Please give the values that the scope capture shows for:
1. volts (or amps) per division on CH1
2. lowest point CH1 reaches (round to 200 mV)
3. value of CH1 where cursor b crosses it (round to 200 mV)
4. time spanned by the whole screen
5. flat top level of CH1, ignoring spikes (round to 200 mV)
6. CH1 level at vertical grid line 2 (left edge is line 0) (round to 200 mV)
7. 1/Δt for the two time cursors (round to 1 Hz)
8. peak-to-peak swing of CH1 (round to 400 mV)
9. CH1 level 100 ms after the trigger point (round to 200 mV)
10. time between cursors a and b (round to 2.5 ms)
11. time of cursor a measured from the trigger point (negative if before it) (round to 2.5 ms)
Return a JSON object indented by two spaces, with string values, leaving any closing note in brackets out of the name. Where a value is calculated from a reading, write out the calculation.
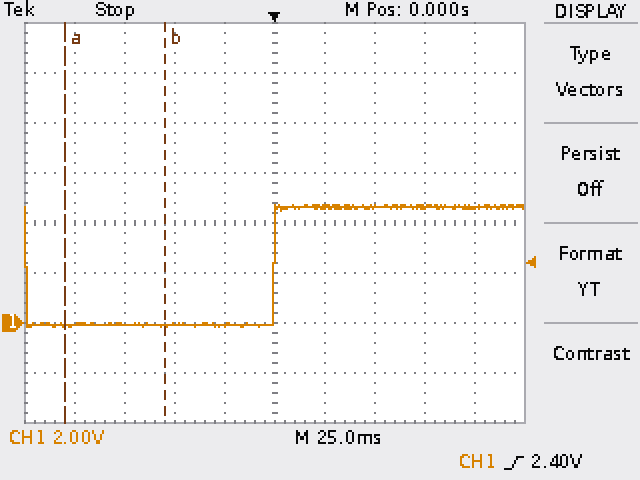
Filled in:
{
  "volts (or amps) per division on CH1": "2 V",
  "lowest point CH1 reaches": "-200 mV",
  "value of CH1 where cursor b crosses it": "-200 mV",
  "time spanned by the whole screen": "250 ms",
  "flat top level of CH1, ignoring spikes": "4.6 V",
  "CH1 level at vertical grid line 2 (left edge is line 0)": "0.0 V",
  "1/Δt for the two time cursors": "1 / 50.0 ms ≈ 20 Hz",
  "peak-to-peak swing of CH1": "4.8 V",
  "CH1 level 100 ms after the trigger point": "4.6 V",
  "time between cursors a and b": "50.0 ms",
  "time of cursor a measured from the trigger point (negative if before it)": "-105.0 ms"
}
